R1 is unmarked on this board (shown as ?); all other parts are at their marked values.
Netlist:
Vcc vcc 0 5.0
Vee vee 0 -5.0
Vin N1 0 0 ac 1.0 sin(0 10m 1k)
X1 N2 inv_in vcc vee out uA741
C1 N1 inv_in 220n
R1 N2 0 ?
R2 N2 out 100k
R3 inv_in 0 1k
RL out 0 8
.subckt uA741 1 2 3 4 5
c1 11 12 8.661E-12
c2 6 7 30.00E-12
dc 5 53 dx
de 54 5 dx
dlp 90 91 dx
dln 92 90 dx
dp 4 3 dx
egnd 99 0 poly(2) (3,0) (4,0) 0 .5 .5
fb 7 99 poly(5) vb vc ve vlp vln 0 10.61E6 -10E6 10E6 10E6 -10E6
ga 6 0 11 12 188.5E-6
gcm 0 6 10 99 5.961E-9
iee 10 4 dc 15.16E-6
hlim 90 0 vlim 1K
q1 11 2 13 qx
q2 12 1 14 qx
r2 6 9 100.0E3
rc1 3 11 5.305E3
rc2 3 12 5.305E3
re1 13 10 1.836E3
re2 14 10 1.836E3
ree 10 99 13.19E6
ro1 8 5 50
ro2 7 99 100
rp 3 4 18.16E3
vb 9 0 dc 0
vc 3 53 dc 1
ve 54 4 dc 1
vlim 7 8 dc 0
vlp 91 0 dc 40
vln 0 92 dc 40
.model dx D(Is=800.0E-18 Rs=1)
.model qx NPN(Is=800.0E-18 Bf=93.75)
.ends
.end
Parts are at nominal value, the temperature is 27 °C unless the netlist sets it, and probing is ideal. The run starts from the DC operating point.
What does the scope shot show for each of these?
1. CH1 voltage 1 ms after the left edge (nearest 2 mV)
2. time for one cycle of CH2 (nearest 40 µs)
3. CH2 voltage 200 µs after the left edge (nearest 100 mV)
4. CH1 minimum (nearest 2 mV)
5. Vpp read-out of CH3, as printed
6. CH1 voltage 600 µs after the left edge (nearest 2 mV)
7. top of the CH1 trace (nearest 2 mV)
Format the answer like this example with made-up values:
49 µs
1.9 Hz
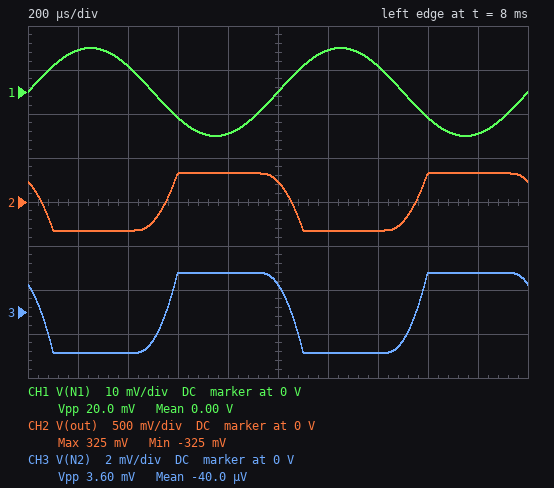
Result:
0 V
1.00 ms
-300 mV
-10 mV
3.60 mV
-6 mV
10 mV
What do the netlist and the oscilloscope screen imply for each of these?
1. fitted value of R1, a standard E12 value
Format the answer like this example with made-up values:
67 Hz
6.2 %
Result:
560 Ω
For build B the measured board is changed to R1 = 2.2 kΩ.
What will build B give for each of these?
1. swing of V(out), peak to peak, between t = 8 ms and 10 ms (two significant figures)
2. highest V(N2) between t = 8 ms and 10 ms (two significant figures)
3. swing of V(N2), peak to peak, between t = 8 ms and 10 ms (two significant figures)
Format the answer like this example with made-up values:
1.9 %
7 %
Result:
650 mV
6.8 mV
14 mV
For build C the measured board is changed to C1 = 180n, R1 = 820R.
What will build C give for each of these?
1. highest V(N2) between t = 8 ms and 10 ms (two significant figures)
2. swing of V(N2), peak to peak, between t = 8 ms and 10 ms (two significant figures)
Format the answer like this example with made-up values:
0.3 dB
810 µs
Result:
2.6 mV
5.3 mV
